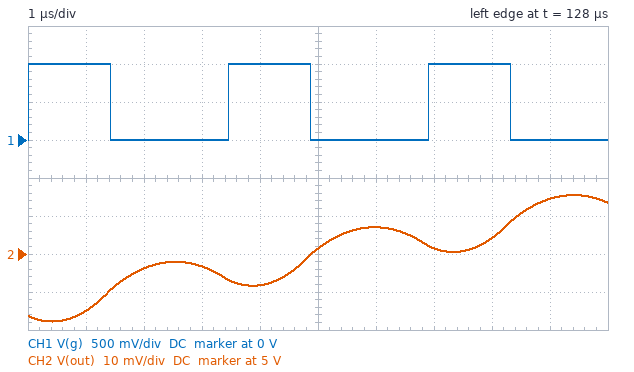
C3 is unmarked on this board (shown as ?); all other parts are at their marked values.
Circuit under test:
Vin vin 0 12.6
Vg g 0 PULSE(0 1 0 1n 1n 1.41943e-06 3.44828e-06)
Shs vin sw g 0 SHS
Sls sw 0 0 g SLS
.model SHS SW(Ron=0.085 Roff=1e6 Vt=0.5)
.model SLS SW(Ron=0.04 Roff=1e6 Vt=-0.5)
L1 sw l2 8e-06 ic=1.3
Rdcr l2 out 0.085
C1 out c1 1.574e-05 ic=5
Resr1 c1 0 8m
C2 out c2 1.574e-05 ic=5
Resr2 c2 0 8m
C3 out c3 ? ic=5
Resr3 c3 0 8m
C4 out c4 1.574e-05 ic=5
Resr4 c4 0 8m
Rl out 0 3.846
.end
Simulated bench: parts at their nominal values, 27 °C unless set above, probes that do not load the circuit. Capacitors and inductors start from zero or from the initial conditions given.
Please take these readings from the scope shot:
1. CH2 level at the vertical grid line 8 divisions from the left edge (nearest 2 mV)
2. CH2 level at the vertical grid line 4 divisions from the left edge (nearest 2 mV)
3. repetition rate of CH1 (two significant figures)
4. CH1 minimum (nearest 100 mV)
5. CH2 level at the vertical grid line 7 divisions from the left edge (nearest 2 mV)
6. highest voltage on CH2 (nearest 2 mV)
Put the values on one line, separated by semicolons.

5.004 V; 4.992 V; 290 kHz; 0 V; 5.002 V; 5.016 V
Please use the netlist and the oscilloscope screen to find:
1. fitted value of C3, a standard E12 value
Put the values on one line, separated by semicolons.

8.2 µF
